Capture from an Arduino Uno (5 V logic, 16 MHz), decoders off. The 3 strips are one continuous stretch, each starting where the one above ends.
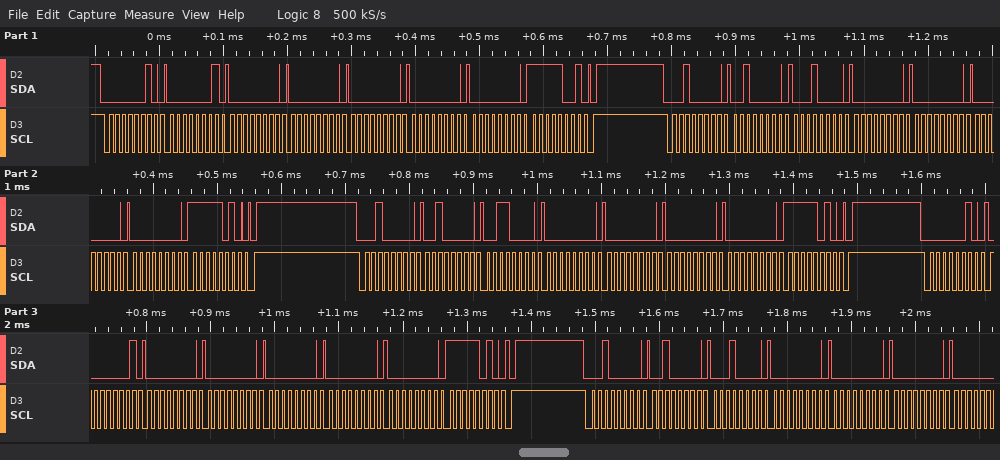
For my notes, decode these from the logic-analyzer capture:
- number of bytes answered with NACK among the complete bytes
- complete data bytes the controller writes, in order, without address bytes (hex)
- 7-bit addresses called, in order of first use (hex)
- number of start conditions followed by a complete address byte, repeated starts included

0
01 00 00 00 00 00 F9 20 10 00 00 00 00 FA 20 30 00 00 00 00 FA 01 00 00 00 00 00 FA 20 10 00 00 00
0x01 0x10
5
